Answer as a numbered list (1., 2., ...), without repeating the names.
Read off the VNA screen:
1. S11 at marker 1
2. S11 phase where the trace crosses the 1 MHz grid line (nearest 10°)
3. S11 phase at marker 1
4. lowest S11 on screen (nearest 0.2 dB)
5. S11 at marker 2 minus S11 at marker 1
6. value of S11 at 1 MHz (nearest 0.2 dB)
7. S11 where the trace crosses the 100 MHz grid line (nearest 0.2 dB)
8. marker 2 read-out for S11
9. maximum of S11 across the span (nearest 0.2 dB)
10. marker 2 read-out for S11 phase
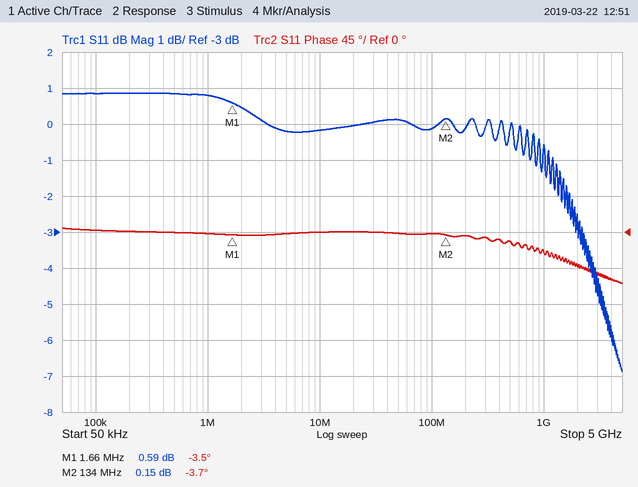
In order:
1. 0.59 dB
2. 0°
3. -3.5°
4. -6.8 dB
5. -0.44 dB
6. 0.8 dB
7. -0.2 dB
8. 0.15 dB
9. 0.8 dB
10. -3.7°
